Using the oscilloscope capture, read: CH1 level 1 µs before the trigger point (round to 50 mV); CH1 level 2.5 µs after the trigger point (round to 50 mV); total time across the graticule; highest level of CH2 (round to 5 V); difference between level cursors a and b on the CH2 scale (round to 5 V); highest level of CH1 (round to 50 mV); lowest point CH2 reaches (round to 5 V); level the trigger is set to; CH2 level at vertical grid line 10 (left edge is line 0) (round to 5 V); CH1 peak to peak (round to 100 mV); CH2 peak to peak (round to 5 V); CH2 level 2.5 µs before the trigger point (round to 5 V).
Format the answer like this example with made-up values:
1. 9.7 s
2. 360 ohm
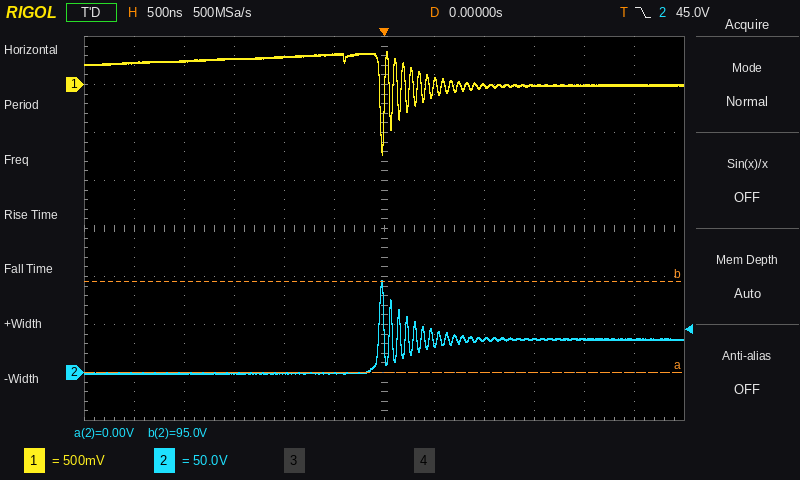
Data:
1. 300 mV
2. 0 mV
3. 6 µs
4. 95 V
5. 95 V
6. 350 mV
7. 0 V
8. 45.0 V
9. 35 V
10. 1.10 V
11. 95 V
12. 0 V
